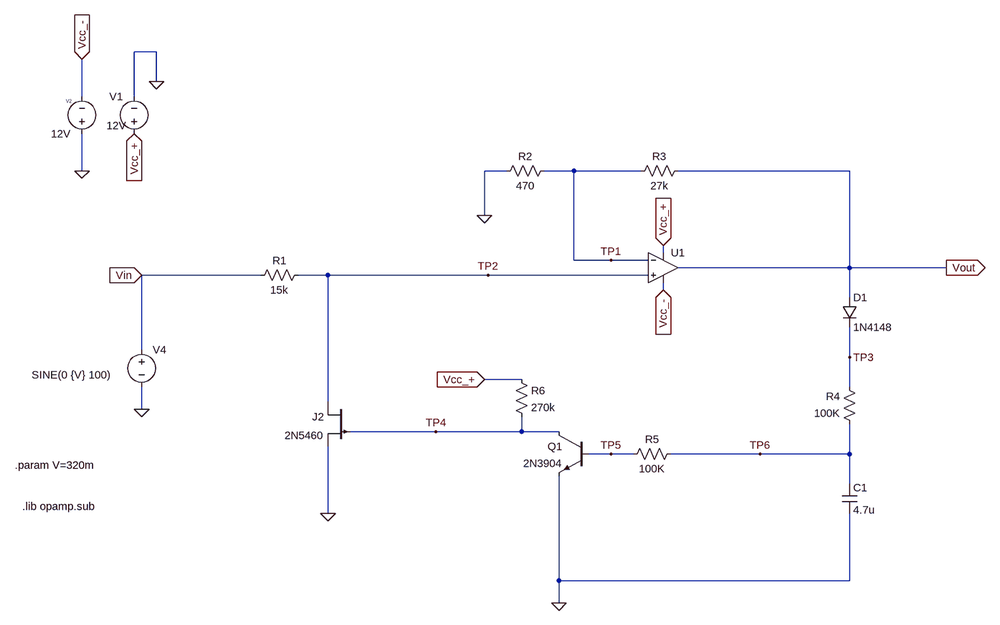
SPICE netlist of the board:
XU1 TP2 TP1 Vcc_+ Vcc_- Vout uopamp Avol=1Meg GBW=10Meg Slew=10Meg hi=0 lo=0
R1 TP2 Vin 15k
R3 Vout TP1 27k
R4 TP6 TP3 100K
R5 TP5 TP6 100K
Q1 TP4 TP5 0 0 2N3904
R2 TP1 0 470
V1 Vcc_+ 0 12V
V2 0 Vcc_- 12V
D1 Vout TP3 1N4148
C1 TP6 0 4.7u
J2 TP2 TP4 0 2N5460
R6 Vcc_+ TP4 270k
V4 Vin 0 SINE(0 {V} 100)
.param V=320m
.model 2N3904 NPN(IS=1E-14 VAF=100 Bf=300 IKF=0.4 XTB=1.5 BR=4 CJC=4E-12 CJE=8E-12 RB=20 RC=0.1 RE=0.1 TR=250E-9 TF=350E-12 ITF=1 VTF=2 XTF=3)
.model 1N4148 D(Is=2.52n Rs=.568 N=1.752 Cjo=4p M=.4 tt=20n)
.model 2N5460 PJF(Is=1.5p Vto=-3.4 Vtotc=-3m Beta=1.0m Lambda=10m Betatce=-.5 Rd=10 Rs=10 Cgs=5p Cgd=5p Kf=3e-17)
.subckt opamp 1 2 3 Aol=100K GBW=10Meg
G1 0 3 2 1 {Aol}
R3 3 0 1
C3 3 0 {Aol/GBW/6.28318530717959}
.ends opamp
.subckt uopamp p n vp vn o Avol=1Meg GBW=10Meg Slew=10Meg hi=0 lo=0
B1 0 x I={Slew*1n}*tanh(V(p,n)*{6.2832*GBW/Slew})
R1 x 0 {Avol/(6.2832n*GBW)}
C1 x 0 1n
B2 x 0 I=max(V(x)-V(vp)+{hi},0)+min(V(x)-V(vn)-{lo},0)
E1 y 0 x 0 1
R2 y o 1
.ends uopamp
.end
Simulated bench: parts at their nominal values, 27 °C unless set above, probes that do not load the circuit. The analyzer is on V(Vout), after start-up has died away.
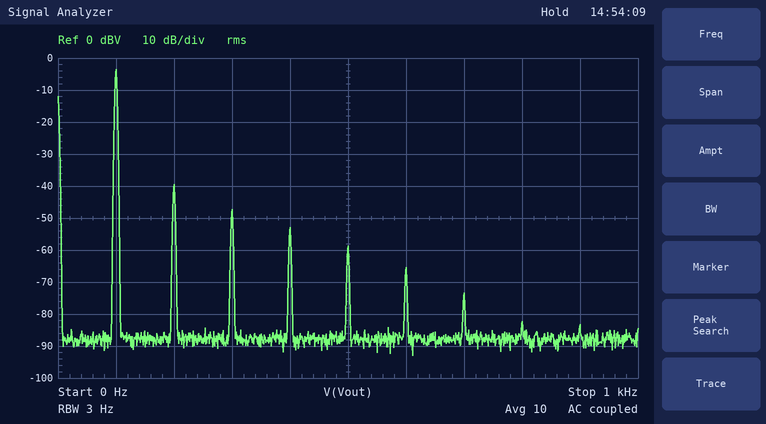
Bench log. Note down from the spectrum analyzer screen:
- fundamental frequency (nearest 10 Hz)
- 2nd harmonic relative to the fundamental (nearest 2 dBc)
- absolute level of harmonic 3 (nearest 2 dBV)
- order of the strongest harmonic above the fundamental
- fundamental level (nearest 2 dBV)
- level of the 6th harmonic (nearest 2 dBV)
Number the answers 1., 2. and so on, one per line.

1. 100 Hz
2. -36 dBc
3. -48 dBV
4. 2
5. -4 dBV
6. -66 dBV
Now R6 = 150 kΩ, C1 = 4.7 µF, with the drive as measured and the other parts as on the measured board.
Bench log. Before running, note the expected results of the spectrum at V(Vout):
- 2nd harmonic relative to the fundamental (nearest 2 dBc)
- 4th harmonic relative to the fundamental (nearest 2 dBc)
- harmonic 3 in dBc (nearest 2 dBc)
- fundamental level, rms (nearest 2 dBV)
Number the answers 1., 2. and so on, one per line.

1. -32 dBc
2. -46 dBc
3. -40 dBc
4. -2 dBV
